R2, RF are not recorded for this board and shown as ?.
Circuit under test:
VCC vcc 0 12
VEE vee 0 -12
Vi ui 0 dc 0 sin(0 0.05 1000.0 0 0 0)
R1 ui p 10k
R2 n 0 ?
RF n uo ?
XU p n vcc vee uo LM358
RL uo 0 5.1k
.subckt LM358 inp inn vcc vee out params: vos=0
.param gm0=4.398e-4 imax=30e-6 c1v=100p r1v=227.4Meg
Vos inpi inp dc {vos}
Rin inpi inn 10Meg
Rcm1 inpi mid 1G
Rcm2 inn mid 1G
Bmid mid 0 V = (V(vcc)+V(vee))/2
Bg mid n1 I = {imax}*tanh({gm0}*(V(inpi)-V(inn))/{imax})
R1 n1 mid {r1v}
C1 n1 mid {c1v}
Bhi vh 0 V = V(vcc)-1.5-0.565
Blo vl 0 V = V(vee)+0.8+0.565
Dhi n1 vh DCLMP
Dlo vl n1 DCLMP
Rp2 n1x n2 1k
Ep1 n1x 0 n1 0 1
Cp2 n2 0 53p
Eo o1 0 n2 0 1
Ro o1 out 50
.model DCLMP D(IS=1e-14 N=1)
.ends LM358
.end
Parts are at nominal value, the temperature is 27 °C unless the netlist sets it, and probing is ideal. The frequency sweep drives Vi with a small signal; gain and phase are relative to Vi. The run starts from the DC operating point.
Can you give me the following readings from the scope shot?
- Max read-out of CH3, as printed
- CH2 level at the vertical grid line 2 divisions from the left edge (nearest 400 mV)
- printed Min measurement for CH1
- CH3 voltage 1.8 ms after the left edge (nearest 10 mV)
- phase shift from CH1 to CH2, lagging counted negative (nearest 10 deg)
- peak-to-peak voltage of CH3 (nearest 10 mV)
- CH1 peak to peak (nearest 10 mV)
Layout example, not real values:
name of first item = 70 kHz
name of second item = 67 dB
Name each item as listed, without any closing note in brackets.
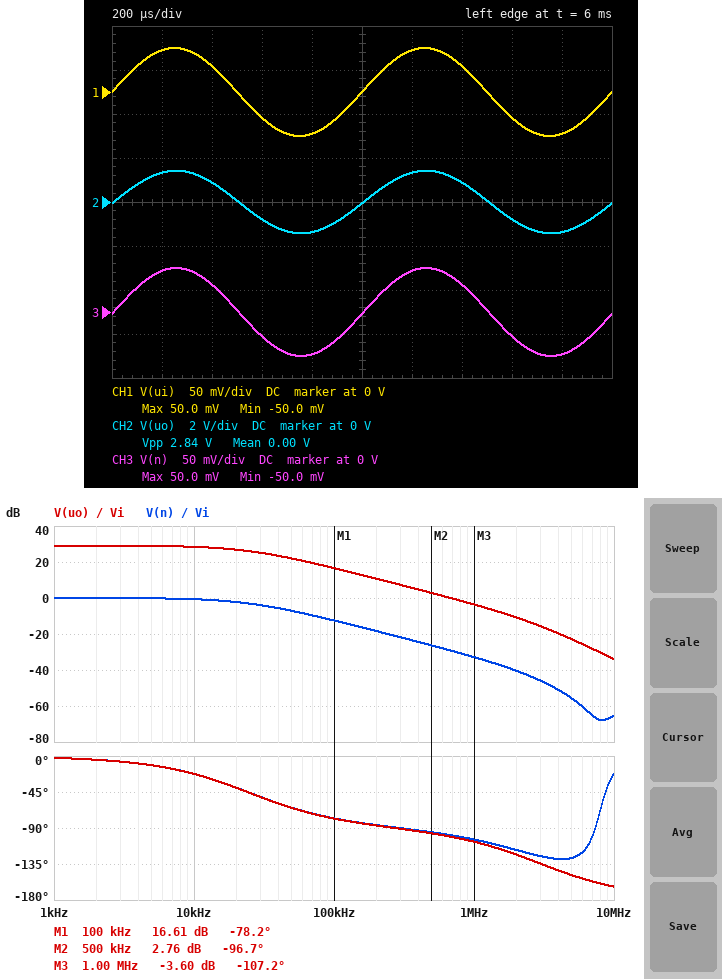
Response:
Max read-out of CH3, as printed = 50.0 mV
CH2 level at the vertical grid line 2 divisions from the left edge = 800 mV
printed Min measurement for CH1 = -50.0 mV
CH3 voltage 1.8 ms after the left edge = -50 mV
phase shift from CH1 to CH2, lagging counted negative = 0 deg
peak-to-peak voltage of CH3 = 100 mV
CH1 peak to peak = 100 mV
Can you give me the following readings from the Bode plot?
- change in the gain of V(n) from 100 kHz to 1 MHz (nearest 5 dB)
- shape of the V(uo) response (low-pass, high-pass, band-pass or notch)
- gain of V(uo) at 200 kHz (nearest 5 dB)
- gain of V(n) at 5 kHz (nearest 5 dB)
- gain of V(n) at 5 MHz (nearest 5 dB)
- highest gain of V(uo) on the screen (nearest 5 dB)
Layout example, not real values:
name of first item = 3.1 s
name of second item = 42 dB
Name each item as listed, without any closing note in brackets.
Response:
change in the gain of V(n) from 100 kHz to 1 MHz = -20 dB
shape of the V(uo) response = low-pass
gain of V(uo) at 200 kHz = 10 dB
gain of V(n) at 5 kHz = 0 dB
gain of V(n) at 5 MHz = -55 dB
highest gain of V(uo) on the screen = 30 dB
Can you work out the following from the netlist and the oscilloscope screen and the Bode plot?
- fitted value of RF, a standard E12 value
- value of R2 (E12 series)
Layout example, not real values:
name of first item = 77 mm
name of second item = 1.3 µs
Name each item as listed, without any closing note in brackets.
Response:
fitted value of RF, a standard E12 value = 330 kΩ
value of R2 = 12 kΩ
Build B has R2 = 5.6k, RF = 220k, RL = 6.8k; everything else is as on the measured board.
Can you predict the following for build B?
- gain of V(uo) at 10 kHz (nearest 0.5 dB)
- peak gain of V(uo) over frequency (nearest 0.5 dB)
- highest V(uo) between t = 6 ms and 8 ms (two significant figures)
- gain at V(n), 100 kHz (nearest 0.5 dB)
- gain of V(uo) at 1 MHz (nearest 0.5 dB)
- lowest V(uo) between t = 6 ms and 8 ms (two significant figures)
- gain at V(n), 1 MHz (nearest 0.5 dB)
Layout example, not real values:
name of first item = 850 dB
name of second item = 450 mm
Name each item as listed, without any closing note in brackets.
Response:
gain of V(uo) at 10 kHz = 31.0 dB
peak gain of V(uo) over frequency = 32.0 dB
highest V(uo) between t = 6 ms and 8 ms = 2.0 V
gain at V(n), 100 kHz = -15.5 dB
gain of V(uo) at 1 MHz = -3.5 dB
lowest V(uo) between t = 6 ms and 8 ms = -2.0 V
gain at V(n), 1 MHz = -36.0 dB
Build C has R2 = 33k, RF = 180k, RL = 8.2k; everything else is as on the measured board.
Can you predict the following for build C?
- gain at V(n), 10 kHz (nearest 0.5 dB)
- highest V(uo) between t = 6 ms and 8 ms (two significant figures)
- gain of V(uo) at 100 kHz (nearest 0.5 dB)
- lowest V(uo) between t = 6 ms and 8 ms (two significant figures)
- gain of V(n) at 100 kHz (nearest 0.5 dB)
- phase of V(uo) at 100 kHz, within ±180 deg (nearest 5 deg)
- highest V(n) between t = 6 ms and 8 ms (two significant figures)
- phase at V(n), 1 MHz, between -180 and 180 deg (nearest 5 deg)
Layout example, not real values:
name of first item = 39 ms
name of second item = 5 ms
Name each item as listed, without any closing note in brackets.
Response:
gain at V(n), 10 kHz = 0 dB
highest V(uo) between t = 6 ms and 8 ms = 320 mV
gain of V(uo) at 100 kHz = 13.5 dB
lowest V(uo) between t = 6 ms and 8 ms = -320 mV
gain of V(n) at 100 kHz = -2.5 dB
phase of V(uo) at 100 kHz, within ±180 deg = -45 deg
highest V(n) between t = 6 ms and 8 ms = 50 mV
phase at V(n), 1 MHz, between -180 and 180 deg = -100 deg
